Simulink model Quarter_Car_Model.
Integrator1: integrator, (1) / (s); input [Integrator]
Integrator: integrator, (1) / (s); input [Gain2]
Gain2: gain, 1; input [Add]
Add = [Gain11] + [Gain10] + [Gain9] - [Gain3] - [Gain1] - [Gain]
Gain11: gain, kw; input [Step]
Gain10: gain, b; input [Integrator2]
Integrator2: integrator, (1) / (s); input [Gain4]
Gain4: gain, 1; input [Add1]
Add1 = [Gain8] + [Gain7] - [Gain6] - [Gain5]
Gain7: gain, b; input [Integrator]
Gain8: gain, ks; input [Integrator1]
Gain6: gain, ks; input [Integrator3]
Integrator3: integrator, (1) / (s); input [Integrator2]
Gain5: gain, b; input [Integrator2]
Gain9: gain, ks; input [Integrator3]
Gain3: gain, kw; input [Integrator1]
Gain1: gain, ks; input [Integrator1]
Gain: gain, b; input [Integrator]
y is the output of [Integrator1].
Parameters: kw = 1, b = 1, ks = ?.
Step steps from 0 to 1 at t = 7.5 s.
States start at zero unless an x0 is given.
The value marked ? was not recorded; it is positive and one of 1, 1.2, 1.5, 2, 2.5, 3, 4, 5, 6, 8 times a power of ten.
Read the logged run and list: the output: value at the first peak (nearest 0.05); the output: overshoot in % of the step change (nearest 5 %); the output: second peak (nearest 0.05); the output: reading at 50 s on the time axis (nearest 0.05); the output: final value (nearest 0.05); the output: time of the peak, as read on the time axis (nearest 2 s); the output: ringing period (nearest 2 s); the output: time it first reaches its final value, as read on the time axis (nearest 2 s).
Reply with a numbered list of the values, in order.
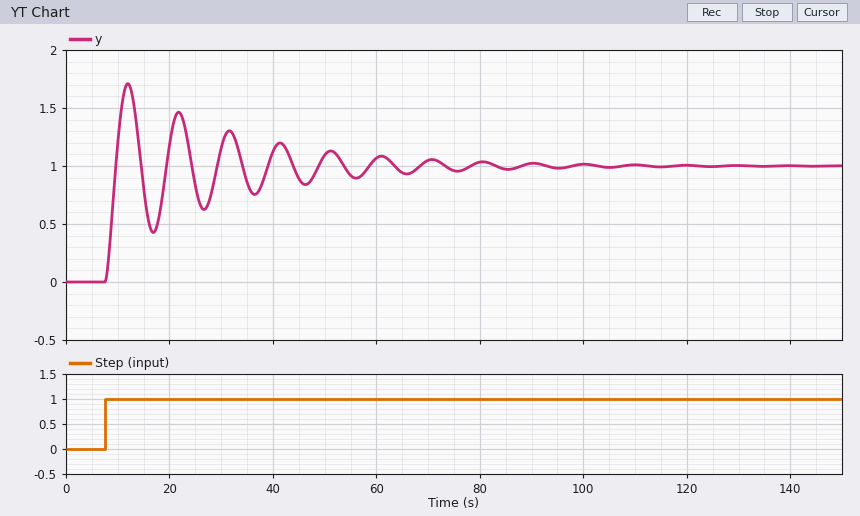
1. 1.70
2. 70 %
3. 1.45
4. 1.10
5. 1.00
6. 12 s
7. 10 s
8. 10 s
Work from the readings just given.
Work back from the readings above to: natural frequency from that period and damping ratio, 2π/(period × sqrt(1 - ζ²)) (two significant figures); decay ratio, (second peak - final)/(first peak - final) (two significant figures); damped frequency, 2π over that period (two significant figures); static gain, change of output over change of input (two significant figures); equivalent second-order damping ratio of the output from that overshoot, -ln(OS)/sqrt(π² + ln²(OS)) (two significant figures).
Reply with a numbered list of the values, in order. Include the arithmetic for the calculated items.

1. 2π / (10 × sqrt(1 - 0.11²)) = 0.63 rad/s
2. (1.45 - 1) / (1.7 - 1) = 0.64
3. 2π / 10 = 0.63 rad/s
4. (1 - 0) / (1 - 0) = 1.0
5. ln(0.7) = -0.357; 0.357 / sqrt(9.870 + 0.127) = 0.11
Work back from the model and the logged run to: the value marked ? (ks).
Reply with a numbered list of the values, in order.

1. 1
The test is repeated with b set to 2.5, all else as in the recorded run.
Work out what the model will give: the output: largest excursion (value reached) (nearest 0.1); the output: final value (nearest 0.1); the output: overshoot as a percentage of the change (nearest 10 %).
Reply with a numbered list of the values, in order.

1. 1.8
2. 1.0
3. 80 %
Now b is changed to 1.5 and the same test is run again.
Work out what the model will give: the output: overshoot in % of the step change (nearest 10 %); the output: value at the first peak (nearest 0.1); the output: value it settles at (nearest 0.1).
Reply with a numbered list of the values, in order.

1. 80 %
2. 1.8
3. 1.0
